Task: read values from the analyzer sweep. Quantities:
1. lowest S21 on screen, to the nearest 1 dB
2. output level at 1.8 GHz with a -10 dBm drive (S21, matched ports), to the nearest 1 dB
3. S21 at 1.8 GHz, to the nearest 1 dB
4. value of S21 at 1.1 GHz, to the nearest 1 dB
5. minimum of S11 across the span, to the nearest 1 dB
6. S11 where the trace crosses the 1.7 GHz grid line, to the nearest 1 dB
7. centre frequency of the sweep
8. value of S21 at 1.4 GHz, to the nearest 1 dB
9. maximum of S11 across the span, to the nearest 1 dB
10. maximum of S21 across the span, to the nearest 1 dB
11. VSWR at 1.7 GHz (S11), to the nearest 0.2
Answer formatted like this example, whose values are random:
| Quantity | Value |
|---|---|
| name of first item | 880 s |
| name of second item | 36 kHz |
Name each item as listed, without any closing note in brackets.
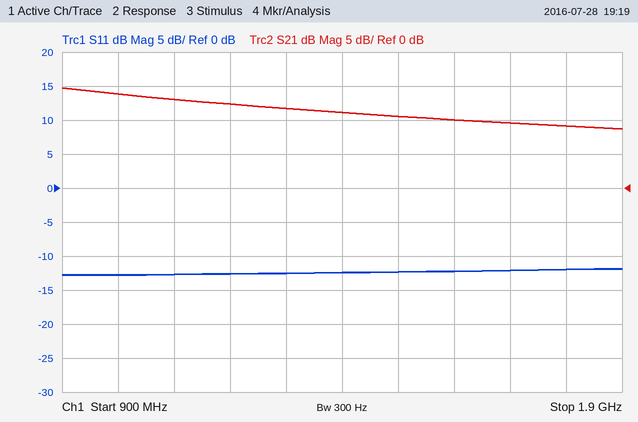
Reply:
| Quantity | Value |
|---|---|
| lowest S21 on screen, to the nearest 1 dB | 9 dB |
| output level at 1.8 GHz with a -10 dBm drive (S21, matched ports), to the nearest 1 dB | -1 dBm |
| S21 at 1.8 GHz, to the nearest 1 dB | 9 dB |
| value of S21 at 1.1 GHz, to the nearest 1 dB | 13 dB |
| minimum of S11 across the span, to the nearest 1 dB | -13 dB |
| S11 where the trace crosses the 1.7 GHz grid line, to the nearest 1 dB | -12 dB |
| centre frequency of the sweep | 1.4 GHz |
| value of S21 at 1.4 GHz, to the nearest 1 dB | 11 dB |
| maximum of S11 across the span, to the nearest 1 dB | -12 dB |
| maximum of S21 across the span, to the nearest 1 dB | 15 dB |
| VSWR at 1.7 GHz (S11), to the nearest 0.2 | 1.6 |
